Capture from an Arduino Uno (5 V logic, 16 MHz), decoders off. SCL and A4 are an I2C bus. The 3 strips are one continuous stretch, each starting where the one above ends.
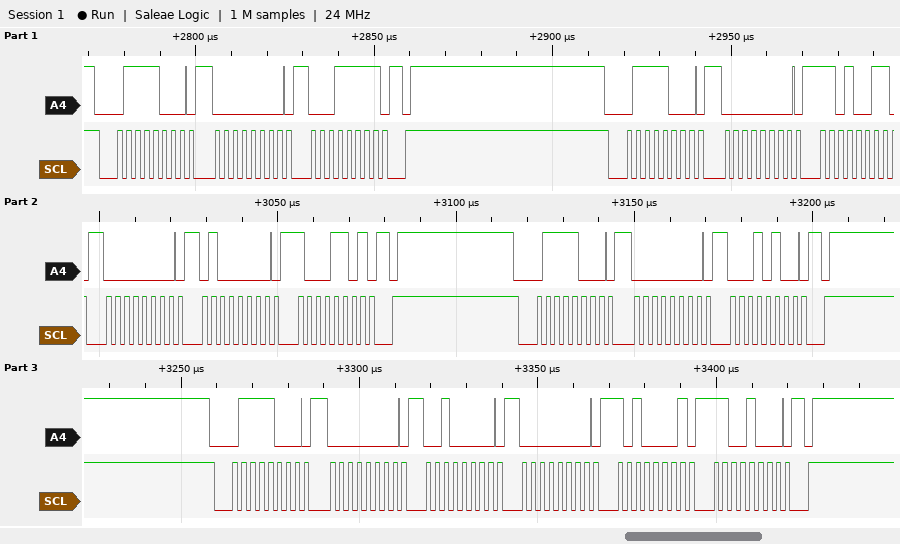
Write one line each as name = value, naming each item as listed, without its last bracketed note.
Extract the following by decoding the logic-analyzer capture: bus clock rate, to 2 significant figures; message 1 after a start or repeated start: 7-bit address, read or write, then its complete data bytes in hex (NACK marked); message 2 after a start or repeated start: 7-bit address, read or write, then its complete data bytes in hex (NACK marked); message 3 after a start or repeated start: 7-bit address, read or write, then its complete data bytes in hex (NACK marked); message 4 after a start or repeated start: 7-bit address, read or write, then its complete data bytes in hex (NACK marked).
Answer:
bus clock rate, to 2 significant figures = 400 kHz
message 1 after a start or repeated start: 7-bit address, read or write, then its complete data bytes in hex = 0x3C write: 00 1F
message 2 after a start or repeated start: 7-bit address, read or write, then its complete data bytes in hex = 0x3C write: 00 D3 00 40 8D
message 3 after a start or repeated start: 7-bit address, read or write, then its complete data bytes in hex = 0x3C write: 00 14
message 4 after a start or repeated start: 7-bit address, read or write, then its complete data bytes in hex = 0x3C write: 00 20 00 A1 C8
